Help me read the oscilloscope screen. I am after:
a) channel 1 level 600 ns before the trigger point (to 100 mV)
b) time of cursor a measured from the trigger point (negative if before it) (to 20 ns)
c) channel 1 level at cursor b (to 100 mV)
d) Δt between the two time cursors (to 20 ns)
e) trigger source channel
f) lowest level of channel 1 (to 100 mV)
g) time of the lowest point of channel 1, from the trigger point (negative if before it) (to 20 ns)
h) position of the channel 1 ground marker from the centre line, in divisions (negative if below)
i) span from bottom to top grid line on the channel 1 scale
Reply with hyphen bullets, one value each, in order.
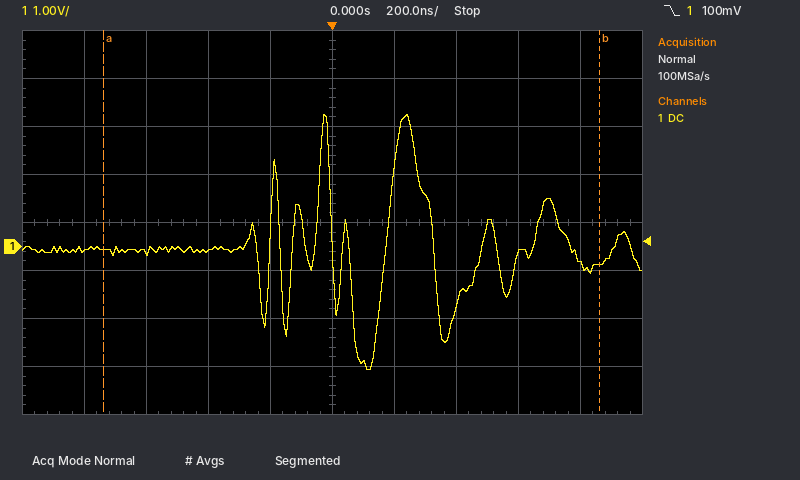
- -100 mV
- -740 ns
- -400 mV
- 1.60 µs
- channel 1
- -2.6 V
- +120 ns
- -0.5 div
- 8 V
